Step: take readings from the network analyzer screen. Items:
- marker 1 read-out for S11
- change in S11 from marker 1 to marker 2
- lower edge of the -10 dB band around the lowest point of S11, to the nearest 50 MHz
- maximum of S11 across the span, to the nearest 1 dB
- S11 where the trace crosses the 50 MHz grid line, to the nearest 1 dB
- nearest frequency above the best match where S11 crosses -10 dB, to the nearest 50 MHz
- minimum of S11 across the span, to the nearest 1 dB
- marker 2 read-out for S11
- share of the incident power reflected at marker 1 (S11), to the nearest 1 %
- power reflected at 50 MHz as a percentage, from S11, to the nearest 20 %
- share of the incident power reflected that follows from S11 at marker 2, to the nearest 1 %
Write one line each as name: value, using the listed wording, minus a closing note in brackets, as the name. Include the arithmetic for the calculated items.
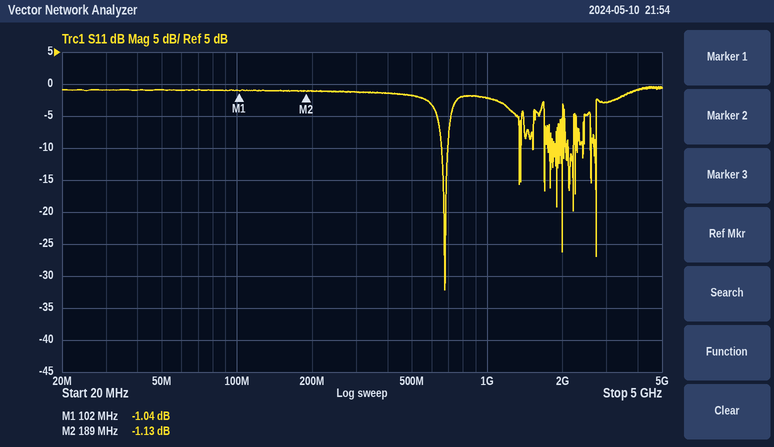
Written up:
marker 1 read-out for S11: -1.04 dB
change in S11 from marker 1 to marker 2: -1.13 − (-1.04) = -0.09 dB
lower edge of the -10 dB band around the lowest point of S11, to the nearest 50 MHz: 650 MHz
maximum of S11 across the span, to the nearest 1 dB: 0 dB
S11 where the trace crosses the 50 MHz grid line, to the nearest 1 dB: -1 dB
nearest frequency above the best match where S11 crosses -10 dB, to the nearest 50 MHz: 700 MHz
minimum of S11 across the span, to the nearest 1 dB: -32 dB
marker 2 read-out for S11: -1.13 dB
share of the incident power reflected at marker 1 (S11), to the nearest 1 %: 10^(-1.04/10) ≈ 79 %
power reflected at 50 MHz as a percentage, from S11, to the nearest 20 %: 10^(-1/10) ≈ 79.4 %, so 80 % to the nearest 20 %
share of the incident power reflected that follows from S11 at marker 2, to the nearest 1 %: 10^(-1.13/10) ≈ 77 %
